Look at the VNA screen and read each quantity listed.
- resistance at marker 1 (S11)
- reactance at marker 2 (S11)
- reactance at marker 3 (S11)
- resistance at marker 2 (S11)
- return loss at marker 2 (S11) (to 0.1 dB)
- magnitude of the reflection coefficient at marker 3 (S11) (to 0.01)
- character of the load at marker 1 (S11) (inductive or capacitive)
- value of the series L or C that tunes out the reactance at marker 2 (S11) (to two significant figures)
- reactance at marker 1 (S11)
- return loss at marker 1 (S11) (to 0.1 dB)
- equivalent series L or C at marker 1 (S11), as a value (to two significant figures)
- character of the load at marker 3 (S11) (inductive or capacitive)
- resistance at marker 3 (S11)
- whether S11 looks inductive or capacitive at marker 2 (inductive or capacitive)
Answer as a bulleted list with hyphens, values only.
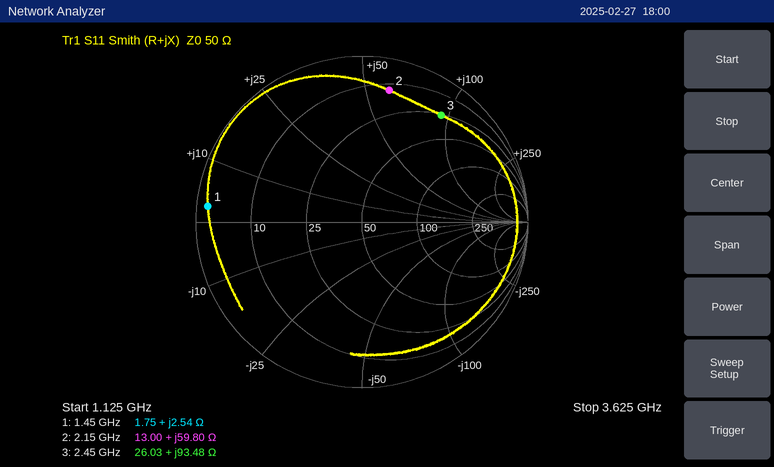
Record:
- 1.75 Ω
- +59.80 Ω
- +93.48 Ω
- 13.00 Ω
- 1.8 dB
- 0.80
- inductive
- 1.2 pF
- +2.54 Ω
- 0.6 dB
- 280 pH
- inductive
- 26.03 Ω
- inductive
